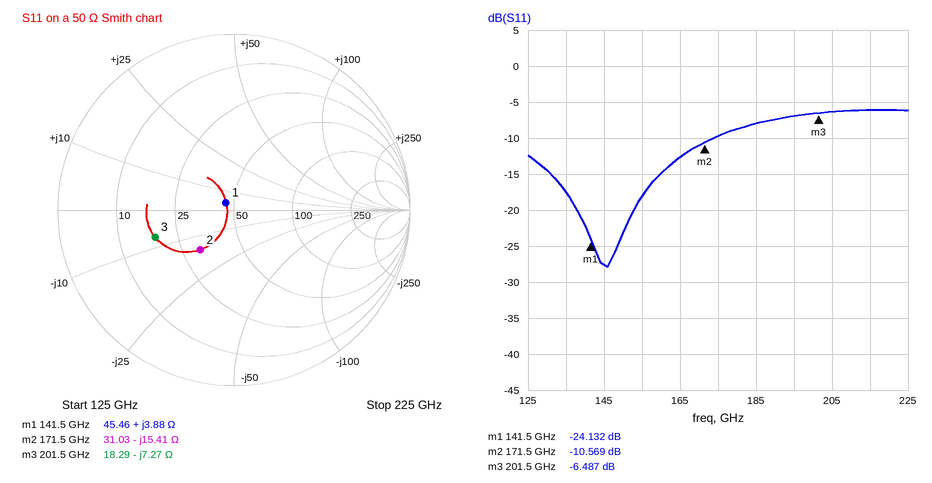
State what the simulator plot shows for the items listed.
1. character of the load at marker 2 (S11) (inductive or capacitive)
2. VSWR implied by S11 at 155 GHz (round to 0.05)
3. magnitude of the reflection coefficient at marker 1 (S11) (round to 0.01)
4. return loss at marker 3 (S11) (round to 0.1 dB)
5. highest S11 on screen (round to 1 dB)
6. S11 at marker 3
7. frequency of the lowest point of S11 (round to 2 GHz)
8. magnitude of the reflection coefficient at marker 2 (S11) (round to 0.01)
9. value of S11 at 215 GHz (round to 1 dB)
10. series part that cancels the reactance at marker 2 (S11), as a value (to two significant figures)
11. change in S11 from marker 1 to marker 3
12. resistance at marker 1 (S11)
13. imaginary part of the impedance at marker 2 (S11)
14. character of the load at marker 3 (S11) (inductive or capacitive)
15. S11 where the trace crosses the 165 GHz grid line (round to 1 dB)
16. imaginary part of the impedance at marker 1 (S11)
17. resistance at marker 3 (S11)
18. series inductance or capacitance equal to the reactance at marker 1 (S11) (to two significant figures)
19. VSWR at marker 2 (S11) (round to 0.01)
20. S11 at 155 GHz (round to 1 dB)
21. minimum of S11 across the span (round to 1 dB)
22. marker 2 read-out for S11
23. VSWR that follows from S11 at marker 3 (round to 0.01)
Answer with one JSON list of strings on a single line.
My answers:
["capacitive", "1.30", "0.06", "6.5 dB", "-6 dB", "-6.487 dB", "146 GHz", "0.30", "-6 dB", "14 pH", "17.645 dB", "45.46 Ω", "-15.41 Ω", "capacitive", "-13 dB", "+3.88 Ω", "18.29 Ω", "4.4 pH", "1.84", "-18 dB", "-28 dB", "-10.569 dB", "2.80"]
